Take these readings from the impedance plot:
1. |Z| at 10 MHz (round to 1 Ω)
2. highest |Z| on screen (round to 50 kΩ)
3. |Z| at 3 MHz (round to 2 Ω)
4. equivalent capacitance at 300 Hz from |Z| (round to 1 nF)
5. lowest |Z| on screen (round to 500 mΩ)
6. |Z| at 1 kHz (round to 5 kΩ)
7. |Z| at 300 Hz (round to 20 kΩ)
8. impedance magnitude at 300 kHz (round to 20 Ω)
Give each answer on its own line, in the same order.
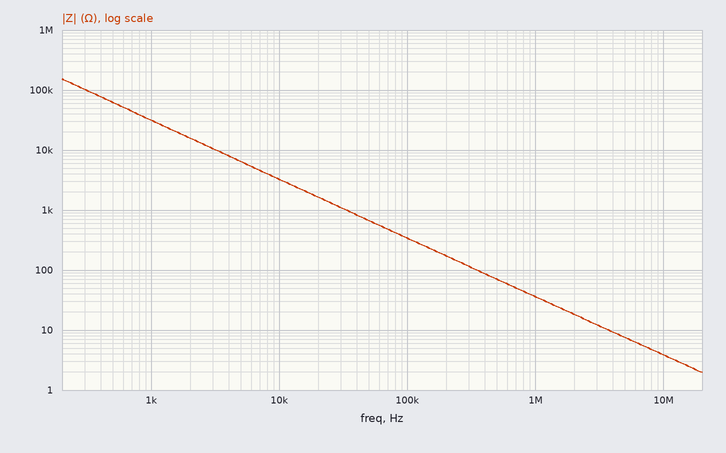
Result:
4 Ω
150 kΩ
12 Ω
5 nF
2.0 Ω
30 kΩ
100 kΩ
120 Ω
